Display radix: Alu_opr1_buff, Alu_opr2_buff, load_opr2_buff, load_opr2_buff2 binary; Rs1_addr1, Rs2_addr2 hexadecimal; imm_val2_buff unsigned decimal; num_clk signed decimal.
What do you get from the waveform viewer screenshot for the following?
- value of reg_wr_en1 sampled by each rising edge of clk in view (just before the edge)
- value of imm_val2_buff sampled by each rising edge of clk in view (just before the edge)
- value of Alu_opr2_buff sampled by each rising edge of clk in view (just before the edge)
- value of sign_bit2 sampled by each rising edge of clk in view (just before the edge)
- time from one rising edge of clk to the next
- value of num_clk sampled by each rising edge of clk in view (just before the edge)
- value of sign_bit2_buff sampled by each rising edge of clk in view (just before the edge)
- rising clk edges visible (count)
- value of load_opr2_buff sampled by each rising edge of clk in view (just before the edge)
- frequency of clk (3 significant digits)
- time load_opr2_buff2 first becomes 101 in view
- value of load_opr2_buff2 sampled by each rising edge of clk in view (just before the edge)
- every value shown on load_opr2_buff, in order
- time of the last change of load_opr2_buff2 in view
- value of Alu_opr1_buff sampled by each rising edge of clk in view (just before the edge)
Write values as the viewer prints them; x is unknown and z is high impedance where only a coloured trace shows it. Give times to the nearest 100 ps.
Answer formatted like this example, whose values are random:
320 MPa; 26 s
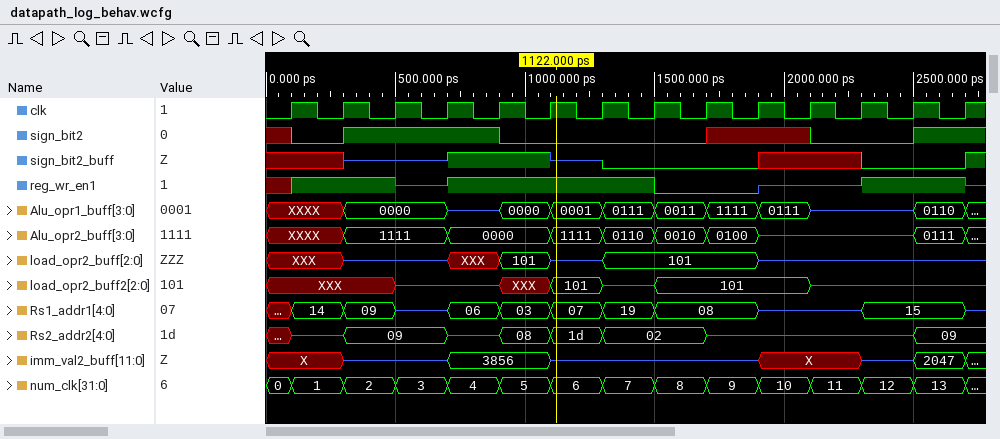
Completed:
x 1 1 z 1 1 1 1 0 0 z z 1 1; X, X, z, z, 3856, 3856, z, z, z, z, X, X, z, 2047; XXXX, XXXX, 1111, 1111, 0000, 0000, 1111, 0110, 0010, 0100, z, z, z, 0111; x 0 1 1 1 0 0 0 0 x x 0 0 1; 200 ps; 0, 1, 2, 3, 4, 5, 6, 7, 8, 9, 10, 11, 12, 13; x x z z 1 1 z 0 0 0 x x 0 0; 14; XXX, XXX, z, z, XXX, 101, z, 101, 101, 101, z, z, z, z; 5.00 GHz; 1100 ps; XXX, XXX, XXX, z, z, XXX, 101, z, 101, 101, 101, z, z, z; XXX, z, XXX, 101, z, 101, z; 2100 ps; XXXX, XXXX, 0000, 0000, z, 0000, 0001, 0111, 0011, 1111, 0111, z, z, 0110
